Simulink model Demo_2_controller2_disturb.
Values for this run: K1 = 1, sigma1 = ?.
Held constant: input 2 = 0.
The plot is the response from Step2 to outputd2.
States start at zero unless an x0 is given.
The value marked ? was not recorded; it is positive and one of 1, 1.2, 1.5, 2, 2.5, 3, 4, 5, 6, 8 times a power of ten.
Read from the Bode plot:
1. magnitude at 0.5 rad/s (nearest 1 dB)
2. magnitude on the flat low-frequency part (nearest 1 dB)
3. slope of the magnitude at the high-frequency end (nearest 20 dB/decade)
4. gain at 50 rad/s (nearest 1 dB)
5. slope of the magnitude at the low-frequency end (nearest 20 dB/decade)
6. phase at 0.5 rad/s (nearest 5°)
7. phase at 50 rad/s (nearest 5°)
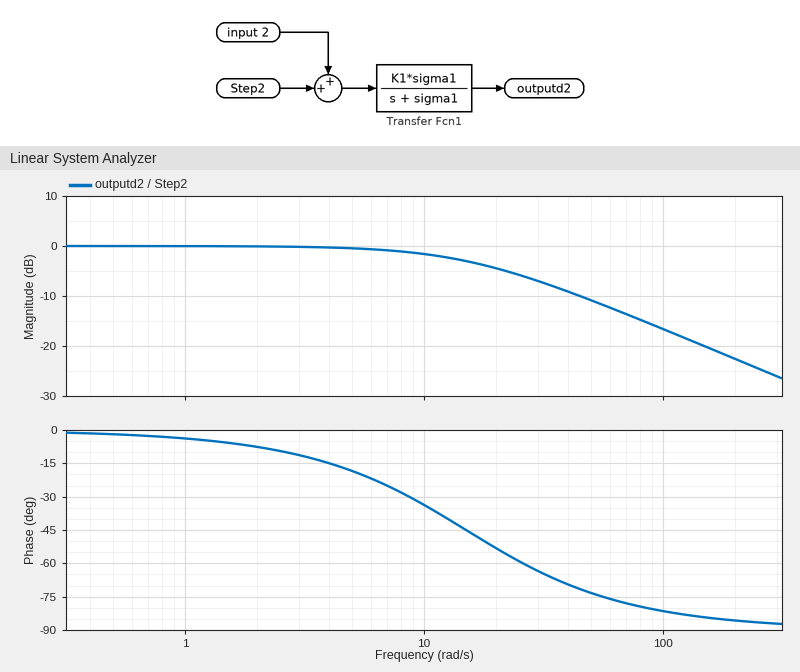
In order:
0 dB
0 dB
-20 dB/decade
-11 dB
0 dB/decade
0°
-75°
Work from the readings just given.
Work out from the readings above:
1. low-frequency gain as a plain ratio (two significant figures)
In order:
1.0
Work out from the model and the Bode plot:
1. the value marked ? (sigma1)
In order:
15
